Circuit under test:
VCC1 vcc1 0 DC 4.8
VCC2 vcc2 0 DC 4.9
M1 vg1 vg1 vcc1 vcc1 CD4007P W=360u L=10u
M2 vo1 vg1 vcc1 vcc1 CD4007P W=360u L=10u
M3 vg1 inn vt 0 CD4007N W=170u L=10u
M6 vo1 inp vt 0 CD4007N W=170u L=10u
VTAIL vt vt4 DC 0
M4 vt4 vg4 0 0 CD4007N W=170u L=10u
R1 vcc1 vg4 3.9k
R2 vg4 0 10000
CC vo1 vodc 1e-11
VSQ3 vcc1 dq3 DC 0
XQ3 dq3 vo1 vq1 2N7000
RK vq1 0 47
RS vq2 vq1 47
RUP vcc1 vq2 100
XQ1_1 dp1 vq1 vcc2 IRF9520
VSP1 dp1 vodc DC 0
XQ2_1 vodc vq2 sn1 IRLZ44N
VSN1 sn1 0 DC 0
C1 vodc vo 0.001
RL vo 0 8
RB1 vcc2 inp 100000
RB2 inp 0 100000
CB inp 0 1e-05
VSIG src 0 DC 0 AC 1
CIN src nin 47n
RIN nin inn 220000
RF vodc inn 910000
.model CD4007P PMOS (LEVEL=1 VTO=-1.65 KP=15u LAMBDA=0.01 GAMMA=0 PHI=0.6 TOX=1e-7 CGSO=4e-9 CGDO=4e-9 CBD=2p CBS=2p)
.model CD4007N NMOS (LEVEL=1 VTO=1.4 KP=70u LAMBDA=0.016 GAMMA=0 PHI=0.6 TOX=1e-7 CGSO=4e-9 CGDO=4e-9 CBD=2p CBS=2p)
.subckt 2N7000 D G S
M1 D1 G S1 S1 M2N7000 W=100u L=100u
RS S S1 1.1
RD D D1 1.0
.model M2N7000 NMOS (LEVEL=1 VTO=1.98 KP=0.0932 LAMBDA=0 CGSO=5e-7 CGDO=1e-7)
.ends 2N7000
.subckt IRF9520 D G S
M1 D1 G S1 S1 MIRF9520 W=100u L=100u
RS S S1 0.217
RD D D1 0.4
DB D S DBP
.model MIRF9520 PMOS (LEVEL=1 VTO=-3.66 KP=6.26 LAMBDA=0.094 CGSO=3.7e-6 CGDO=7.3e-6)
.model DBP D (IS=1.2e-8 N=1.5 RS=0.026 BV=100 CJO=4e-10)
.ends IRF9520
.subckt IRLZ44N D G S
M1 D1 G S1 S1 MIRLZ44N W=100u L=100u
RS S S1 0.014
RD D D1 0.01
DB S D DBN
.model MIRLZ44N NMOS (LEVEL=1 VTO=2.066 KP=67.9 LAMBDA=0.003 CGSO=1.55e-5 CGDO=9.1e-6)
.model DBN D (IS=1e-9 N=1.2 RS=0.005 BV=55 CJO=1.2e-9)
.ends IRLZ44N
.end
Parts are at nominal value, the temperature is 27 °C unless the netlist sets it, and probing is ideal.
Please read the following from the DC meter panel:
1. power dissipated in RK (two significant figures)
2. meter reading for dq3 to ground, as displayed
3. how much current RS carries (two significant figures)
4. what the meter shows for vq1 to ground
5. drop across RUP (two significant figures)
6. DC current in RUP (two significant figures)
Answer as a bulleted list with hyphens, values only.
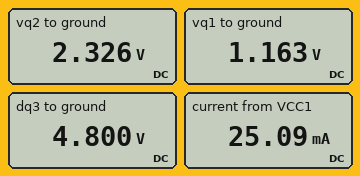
- 29 mW
- 4.800 V
- 25 mA
- 1.163 V
- 2.5 V
- 25 mA
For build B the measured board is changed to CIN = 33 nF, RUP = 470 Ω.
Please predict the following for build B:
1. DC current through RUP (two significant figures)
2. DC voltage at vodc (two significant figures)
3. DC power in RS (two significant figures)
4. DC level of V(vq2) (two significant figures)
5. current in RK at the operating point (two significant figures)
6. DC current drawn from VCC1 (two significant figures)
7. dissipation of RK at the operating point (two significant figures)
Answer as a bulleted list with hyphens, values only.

- 5.8 mA
- 3.5 V
- 1.6 mW
- 2.1 V
- 38 mA
- 40 mA
- 68 mW
